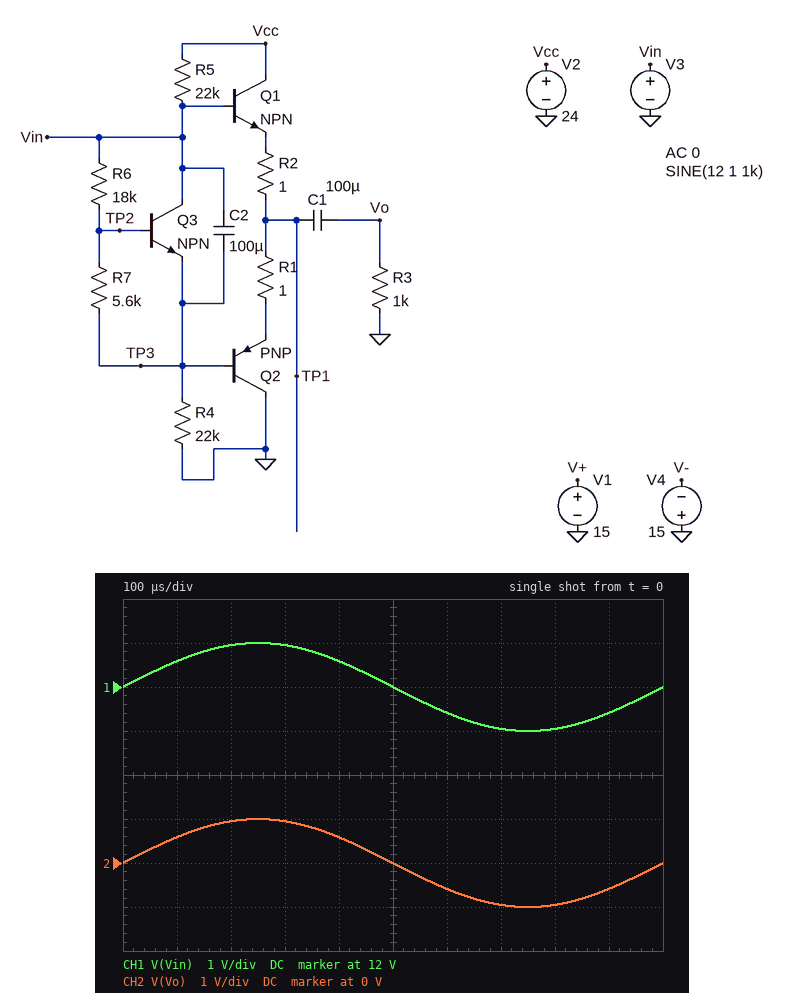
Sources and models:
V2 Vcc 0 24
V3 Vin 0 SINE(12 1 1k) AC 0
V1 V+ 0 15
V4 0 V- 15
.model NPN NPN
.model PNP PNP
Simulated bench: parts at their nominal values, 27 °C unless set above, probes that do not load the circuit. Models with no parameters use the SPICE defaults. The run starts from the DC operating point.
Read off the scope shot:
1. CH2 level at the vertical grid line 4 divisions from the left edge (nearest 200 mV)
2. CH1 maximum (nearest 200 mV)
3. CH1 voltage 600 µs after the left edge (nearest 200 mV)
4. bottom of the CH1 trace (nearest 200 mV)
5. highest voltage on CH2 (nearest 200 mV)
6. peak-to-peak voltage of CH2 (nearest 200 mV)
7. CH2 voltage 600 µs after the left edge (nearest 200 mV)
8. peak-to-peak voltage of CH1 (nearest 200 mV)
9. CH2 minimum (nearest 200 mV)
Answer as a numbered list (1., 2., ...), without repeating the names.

1. 600 mV
2. 13.0 V
3. 11.4 V
4. 11.0 V
5. 1.0 V
6. 2.0 V
7. -600 mV
8. 2.0 V
9. -1.0 V
